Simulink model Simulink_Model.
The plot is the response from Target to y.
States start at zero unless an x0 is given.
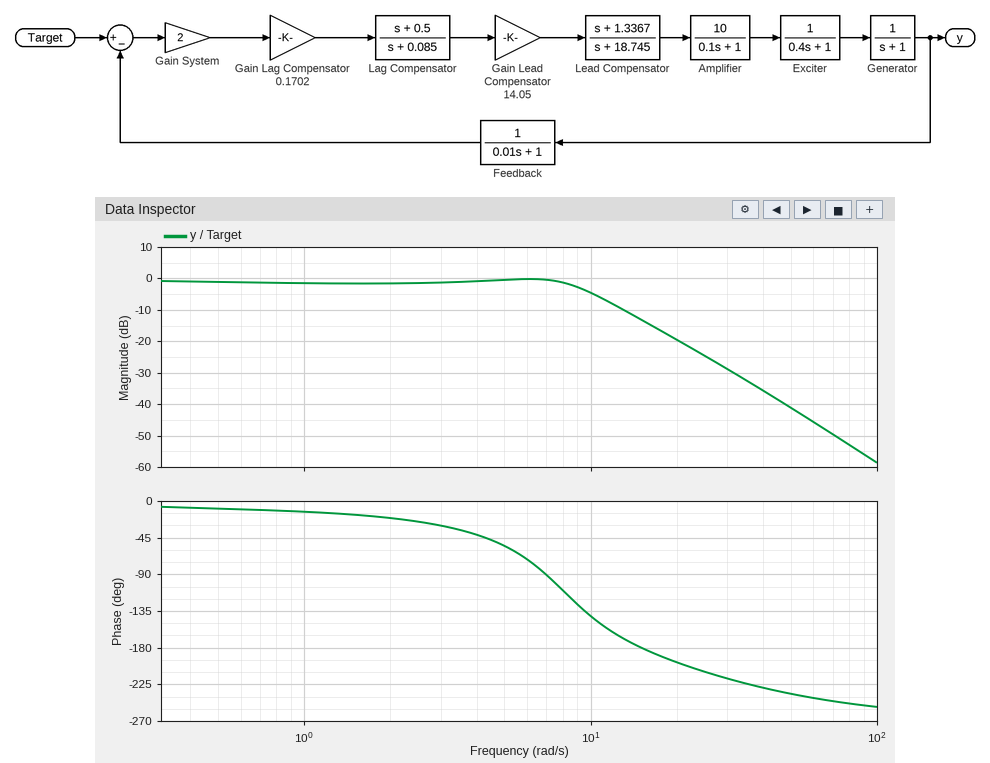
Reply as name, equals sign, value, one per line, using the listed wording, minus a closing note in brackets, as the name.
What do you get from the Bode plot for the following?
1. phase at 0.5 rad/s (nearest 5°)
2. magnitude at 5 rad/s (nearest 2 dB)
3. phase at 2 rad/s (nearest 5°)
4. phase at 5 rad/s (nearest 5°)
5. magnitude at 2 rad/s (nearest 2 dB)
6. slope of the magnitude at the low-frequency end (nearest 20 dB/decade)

phase at 0.5 rad/s = -10°
magnitude at 5 rad/s = 0 dB
phase at 2 rad/s = -20°
phase at 5 rad/s = -55°
magnitude at 2 rad/s = -2 dB
slope of the magnitude at the low-frequency end = 0 dB/decade
